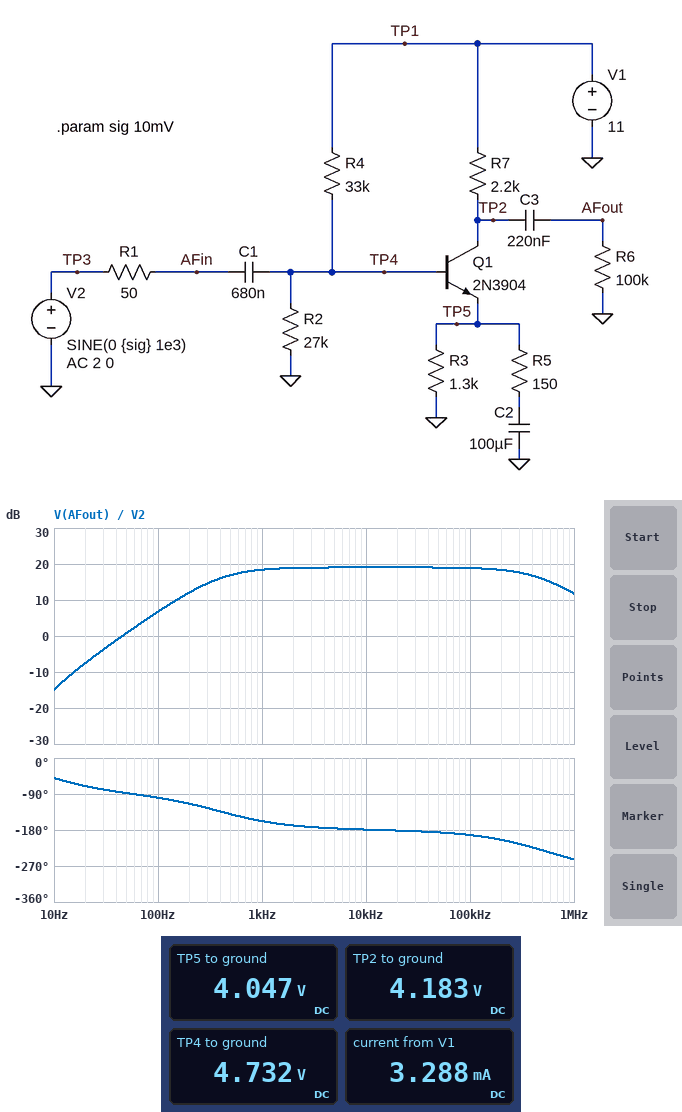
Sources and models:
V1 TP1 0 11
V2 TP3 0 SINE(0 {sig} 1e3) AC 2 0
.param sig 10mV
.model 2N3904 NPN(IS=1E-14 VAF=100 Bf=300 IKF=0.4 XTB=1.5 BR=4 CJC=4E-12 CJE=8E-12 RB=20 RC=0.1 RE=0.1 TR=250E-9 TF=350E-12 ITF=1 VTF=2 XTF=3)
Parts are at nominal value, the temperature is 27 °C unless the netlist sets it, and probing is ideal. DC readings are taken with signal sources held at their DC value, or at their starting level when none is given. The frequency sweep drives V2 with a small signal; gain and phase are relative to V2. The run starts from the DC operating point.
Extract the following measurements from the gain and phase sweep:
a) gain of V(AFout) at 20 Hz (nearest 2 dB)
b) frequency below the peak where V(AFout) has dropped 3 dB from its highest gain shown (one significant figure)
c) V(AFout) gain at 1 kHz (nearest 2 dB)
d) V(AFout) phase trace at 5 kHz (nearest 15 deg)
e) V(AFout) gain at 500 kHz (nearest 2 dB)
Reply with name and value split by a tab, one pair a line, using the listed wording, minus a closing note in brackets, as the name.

gain of V(AFout) at 20 Hz	-8 dB
frequency below the peak where V(AFout) has dropped 3 dB from its highest gain shown	400 Hz
V(AFout) gain at 1 kHz	18 dB
V(AFout) phase trace at 5 kHz	-180 deg
V(AFout) gain at 500 kHz	16 dB
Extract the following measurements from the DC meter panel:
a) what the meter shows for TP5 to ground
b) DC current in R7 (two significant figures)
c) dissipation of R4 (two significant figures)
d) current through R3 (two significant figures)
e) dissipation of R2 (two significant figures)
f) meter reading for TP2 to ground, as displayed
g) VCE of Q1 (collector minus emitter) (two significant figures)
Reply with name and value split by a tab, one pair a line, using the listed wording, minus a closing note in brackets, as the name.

what the meter shows for TP5 to ground	4.047 V
DC current in R7	3.1 mA
dissipation of R4	1.2 mW
current through R3	3.1 mA
dissipation of R2	830 µW
meter reading for TP2 to ground, as displayed	4.183 V
VCE of Q1 (collector minus emitter)	140 mV
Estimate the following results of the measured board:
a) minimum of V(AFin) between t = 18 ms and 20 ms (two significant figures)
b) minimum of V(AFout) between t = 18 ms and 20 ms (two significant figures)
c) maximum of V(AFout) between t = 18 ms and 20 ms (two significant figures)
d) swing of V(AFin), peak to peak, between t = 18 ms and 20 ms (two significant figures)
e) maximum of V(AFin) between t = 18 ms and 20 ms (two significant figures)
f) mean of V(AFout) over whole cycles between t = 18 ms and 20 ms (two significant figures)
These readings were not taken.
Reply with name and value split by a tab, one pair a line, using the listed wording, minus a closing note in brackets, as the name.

minimum of V(AFin) between t = 18 ms and 20 ms	-9.7 mV
minimum of V(AFout) between t = 18 ms and 20 ms	-72 mV
maximum of V(AFout) between t = 18 ms and 20 ms	150 mV
swing of V(AFin), peak to peak, between t = 18 ms and 20 ms	19 mV
maximum of V(AFin) between t = 18 ms and 20 ms	9.4 mV
mean of V(AFout) over whole cycles between t = 18 ms and 20 ms	24 mV
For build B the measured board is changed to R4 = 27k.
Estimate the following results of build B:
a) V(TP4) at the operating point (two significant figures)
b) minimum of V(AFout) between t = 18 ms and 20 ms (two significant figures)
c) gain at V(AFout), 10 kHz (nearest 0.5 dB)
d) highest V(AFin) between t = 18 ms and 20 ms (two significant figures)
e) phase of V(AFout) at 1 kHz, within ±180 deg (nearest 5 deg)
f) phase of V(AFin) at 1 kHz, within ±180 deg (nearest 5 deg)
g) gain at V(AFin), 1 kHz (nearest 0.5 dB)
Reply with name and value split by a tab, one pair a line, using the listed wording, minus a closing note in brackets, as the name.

V(TP4) at the operating point	4.8 V
minimum of V(AFout) between t = 18 ms and 20 ms	-9.6 mV
gain at V(AFout), 10 kHz	3.5 dB
highest V(AFin) between t = 18 ms and 20 ms	9.0 mV
phase of V(AFout) at 1 kHz, within ±180 deg	-140 deg
phase of V(AFin) at 1 kHz, within ±180 deg	-5 deg
gain at V(AFin), 1 kHz	-1.0 dB
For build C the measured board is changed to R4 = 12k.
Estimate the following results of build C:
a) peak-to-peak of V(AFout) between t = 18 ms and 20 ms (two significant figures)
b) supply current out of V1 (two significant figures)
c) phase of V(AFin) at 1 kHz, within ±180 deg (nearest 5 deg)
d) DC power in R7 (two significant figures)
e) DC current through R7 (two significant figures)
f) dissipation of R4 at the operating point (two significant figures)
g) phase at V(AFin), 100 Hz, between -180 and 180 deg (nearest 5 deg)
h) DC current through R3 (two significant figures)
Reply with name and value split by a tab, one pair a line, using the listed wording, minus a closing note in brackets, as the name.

peak-to-peak of V(AFout) between t = 18 ms and 20 ms	4.3 mV
supply current out of V1	3.5 mA
phase of V(AFin) at 1 kHz, within ±180 deg	-5 deg
DC power in R7	20 mW
DC current through R7	3.0 mA
dissipation of R4 at the operating point	3.0 mW
phase at V(AFin), 100 Hz, between -180 and 180 deg	0 deg
DC current through R3	3.3 mA
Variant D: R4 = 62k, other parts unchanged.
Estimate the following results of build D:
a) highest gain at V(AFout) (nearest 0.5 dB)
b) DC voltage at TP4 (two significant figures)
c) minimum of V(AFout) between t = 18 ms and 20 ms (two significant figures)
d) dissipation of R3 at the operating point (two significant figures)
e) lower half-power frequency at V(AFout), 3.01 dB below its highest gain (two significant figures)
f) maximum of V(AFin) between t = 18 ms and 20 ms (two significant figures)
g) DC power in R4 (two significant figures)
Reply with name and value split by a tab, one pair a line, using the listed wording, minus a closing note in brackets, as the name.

highest gain at V(AFout)	23.0 dB
DC voltage at TP4	3.2 V
minimum of V(AFout) between t = 18 ms and 20 ms	-140 mV
dissipation of R3 at the operating point	5.0 mW
lower half-power frequency at V(AFout), 3.01 dB below its highest gain	25 Hz
maximum of V(AFin) between t = 18 ms and 20 ms	10 mV
DC power in R4	980 µW
